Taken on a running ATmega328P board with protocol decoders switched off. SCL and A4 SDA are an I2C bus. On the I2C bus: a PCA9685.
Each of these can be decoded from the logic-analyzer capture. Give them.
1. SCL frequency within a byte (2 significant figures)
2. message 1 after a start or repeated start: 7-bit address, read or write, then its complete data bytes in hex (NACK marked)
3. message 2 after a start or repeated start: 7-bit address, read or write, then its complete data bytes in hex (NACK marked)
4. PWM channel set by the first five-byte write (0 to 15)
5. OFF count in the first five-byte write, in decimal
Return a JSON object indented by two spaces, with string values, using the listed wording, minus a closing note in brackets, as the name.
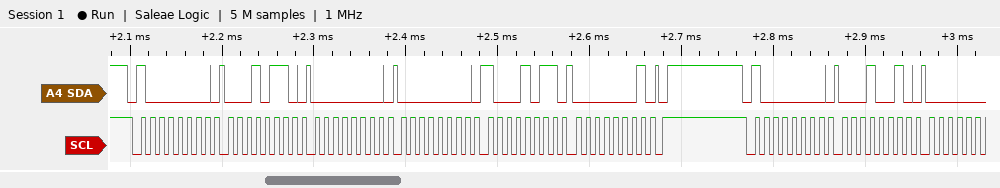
{
  "SCL frequency within a byte": "100 kHz",
  "message 1 after a start or repeated start: 7-bit address, read or write, then its complete data bytes in hex": "0x40 write: 16 00 00 8B 01",
  "message 2 after a start or repeated start: 7-bit address, read or write, then its complete data bytes in hex": "0x40 write: 12",
  "PWM channel set by the first five-byte write": "4",
  "OFF count in the first five-byte write, in decimal": "395"
}
